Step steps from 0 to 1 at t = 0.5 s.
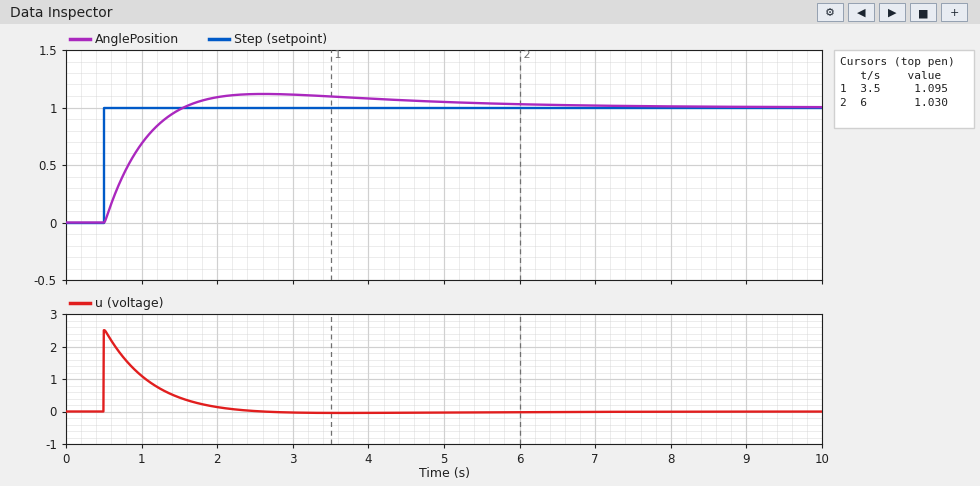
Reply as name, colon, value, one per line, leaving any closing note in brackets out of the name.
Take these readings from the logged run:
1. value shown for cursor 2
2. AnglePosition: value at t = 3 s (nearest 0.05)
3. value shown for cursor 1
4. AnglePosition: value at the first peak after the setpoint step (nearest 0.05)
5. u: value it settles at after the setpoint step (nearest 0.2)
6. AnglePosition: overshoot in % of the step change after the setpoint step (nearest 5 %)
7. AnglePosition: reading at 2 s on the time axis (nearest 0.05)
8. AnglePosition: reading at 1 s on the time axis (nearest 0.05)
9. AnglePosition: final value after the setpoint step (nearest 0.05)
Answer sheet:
value shown for cursor 2: 1.030
AnglePosition: value at t = 3 s: 1.10
value shown for cursor 1: 1.095
AnglePosition: value at the first peak after the setpoint step: 1.10
u: value it settles at after the setpoint step: 0.0
AnglePosition: overshoot in % of the step change after the setpoint step: 10 %
AnglePosition: reading at 2 s on the time axis: 1.10
AnglePosition: reading at 1 s on the time axis: 0.70
AnglePosition: final value after the setpoint step: 1.00
